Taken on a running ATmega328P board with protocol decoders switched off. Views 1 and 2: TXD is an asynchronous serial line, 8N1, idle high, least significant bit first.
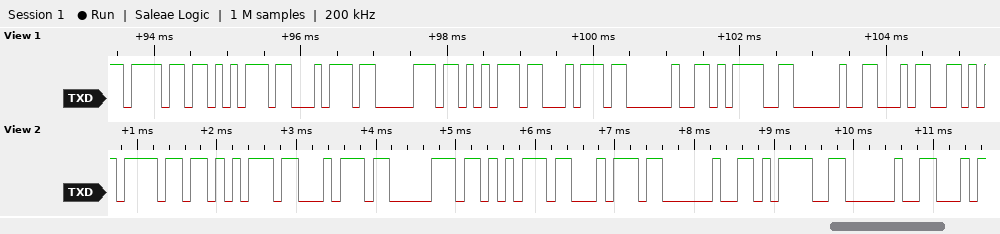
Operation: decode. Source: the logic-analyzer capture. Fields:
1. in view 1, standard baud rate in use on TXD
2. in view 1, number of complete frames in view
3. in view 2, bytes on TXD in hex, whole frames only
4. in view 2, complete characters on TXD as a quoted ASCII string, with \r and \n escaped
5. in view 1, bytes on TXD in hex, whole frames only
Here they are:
9600 baud
10
6F 75 74 70 75 74 20 3D 20
"output = "
6F 75 74 70 75 74 20 3D 20 34
